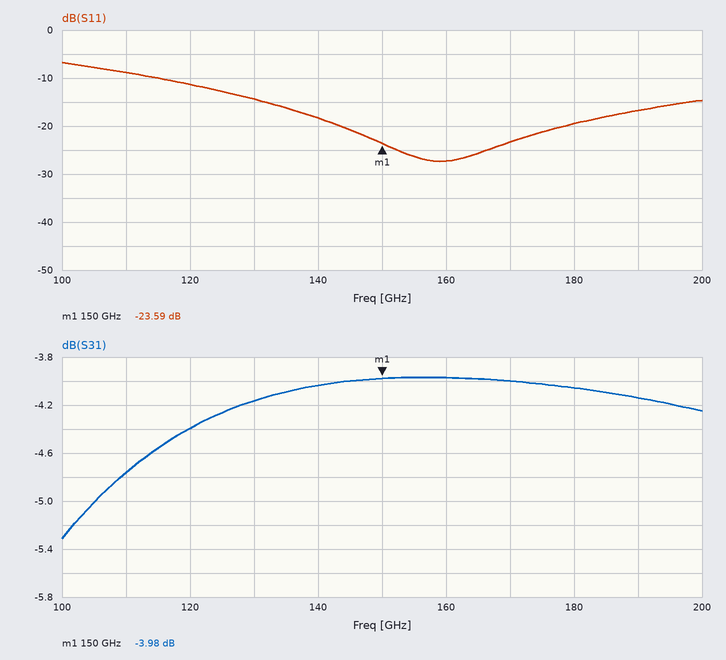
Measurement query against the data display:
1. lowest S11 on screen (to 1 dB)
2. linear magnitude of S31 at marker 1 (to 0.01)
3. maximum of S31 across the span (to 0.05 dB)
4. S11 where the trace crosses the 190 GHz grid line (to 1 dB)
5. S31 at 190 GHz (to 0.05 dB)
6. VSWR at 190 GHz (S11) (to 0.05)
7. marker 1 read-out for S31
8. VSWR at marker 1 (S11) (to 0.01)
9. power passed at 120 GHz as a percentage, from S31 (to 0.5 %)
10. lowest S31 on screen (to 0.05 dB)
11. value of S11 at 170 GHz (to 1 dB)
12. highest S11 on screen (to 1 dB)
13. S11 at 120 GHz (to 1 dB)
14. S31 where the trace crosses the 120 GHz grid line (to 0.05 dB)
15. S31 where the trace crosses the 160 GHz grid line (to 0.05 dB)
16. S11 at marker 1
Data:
-27 dB
0.63
-3.95 dB
-17 dB
-4.15 dB
1.35
-3.98 dB
1.14
36.5 %
-5.30 dB
-23 dB
-7 dB
-11 dB
-4.40 dB
-3.95 dB
-23.59 dB
